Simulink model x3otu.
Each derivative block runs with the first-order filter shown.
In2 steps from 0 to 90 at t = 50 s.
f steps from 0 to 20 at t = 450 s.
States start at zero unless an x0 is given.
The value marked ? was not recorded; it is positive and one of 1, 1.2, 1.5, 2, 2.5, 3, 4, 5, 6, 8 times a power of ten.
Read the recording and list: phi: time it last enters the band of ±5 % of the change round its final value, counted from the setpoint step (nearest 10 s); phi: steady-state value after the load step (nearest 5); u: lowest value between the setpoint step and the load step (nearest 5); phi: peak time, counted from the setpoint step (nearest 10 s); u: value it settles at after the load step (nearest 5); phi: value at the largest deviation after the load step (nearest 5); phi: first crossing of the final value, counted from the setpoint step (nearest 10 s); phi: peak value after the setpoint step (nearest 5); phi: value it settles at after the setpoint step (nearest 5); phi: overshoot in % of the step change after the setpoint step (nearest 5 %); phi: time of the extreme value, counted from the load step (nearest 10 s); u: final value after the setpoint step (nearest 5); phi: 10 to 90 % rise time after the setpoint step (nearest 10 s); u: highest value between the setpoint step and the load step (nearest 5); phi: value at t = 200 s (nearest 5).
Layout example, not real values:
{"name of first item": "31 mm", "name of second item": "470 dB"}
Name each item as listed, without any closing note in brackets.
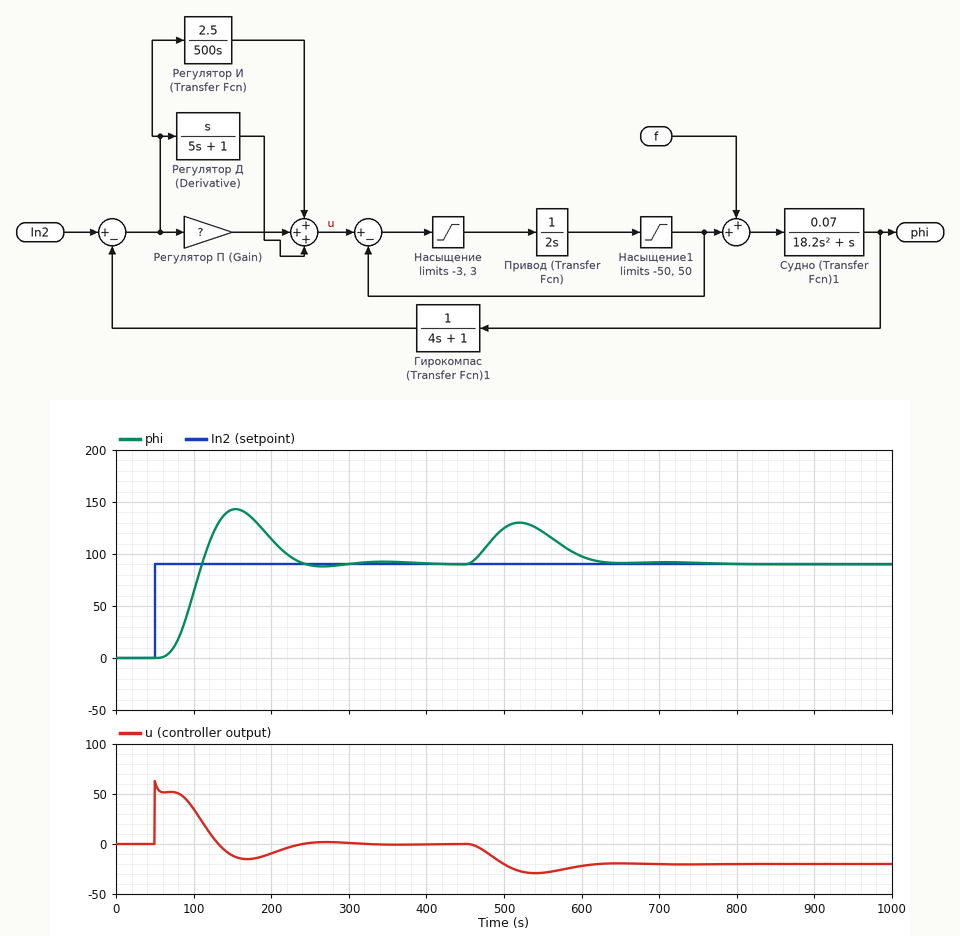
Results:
{"phi: time it last enters the band of ±5 % of the change round its final value, counted from the setpoint step": "180 s", "phi: steady-state value after the load step": "90", "u: lowest value between the setpoint step and the load step": "-15", "phi: peak time, counted from the setpoint step": "100 s", "u: value it settles at after the load step": "-20", "phi: value at the largest deviation after the load step": "130", "phi: first crossing of the final value, counted from the setpoint step": "60 s", "phi: peak value after the setpoint step": "145", "phi: value it settles at after the setpoint step": "90", "phi: overshoot in % of the step change after the setpoint step": "60 %", "phi: time of the extreme value, counted from the load step": "70 s", "u: final value after the setpoint step": "0", "phi: 10 to 90 % rise time after the setpoint step": "30 s", "u: highest value between the setpoint step and the load step": "65", "phi: value at t = 200 s": "115"}
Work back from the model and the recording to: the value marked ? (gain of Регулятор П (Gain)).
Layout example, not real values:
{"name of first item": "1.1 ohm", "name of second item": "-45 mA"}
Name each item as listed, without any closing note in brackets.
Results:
{"the value marked ? (gain of Регулятор П (Gain))": "0.5"}
